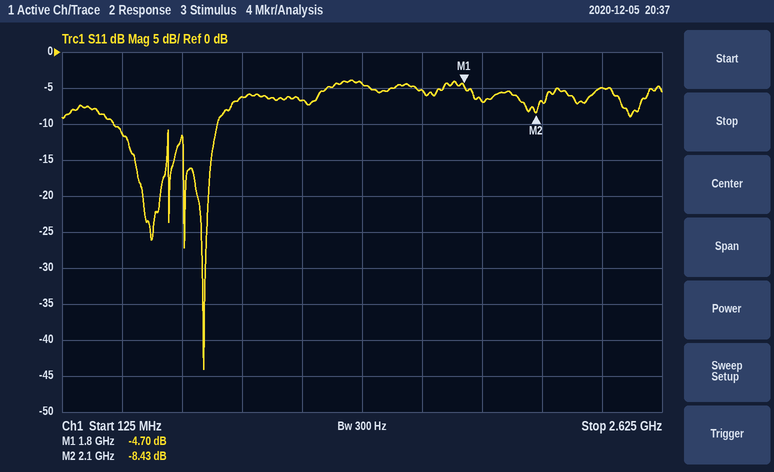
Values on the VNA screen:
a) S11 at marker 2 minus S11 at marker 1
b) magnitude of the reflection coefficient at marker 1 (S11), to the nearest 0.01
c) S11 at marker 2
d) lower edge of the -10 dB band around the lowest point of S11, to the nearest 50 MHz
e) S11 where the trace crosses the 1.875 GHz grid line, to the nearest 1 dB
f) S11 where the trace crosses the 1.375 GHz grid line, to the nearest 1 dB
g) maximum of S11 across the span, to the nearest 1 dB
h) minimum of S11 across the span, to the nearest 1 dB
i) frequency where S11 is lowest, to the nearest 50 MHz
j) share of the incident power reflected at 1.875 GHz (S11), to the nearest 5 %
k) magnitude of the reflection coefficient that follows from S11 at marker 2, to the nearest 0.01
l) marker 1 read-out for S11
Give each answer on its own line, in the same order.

-3.73 dB
0.58
-8.43 dB
350 MHz
-7 dB
-4 dB
-4 dB
-44 dB
700 MHz
20 %
0.38
-4.70 dB
